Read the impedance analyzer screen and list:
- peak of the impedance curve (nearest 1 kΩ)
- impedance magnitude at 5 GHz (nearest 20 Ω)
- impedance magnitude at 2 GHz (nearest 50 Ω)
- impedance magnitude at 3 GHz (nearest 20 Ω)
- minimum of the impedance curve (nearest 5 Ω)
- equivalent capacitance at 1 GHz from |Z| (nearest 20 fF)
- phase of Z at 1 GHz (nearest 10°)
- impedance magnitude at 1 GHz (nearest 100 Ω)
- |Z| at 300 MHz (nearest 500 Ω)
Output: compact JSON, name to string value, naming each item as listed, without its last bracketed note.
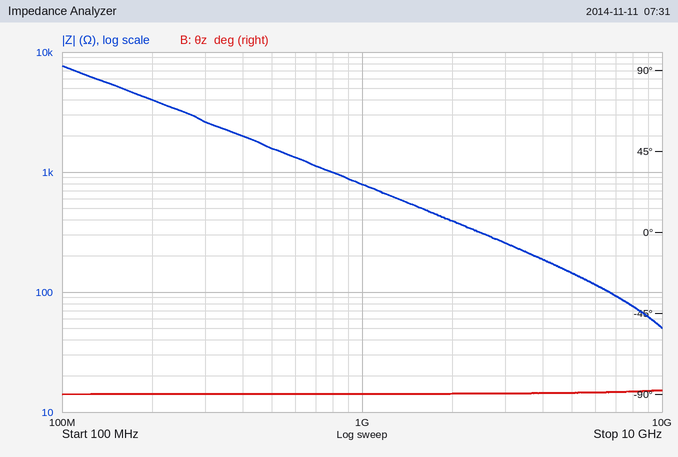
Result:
{"peak of the impedance curve": "8 kΩ", "impedance magnitude at 5 GHz": "140 Ω", "impedance magnitude at 2 GHz": "400 Ω", "impedance magnitude at 3 GHz": "260 Ω", "minimum of the impedance curve": "50 Ω", "equivalent capacitance at 1 GHz from |Z|": "200 fF", "phase of Z at 1 GHz": "-90°", "impedance magnitude at 1 GHz": "800 Ω", "|Z| at 300 MHz": "2.5 kΩ"}
